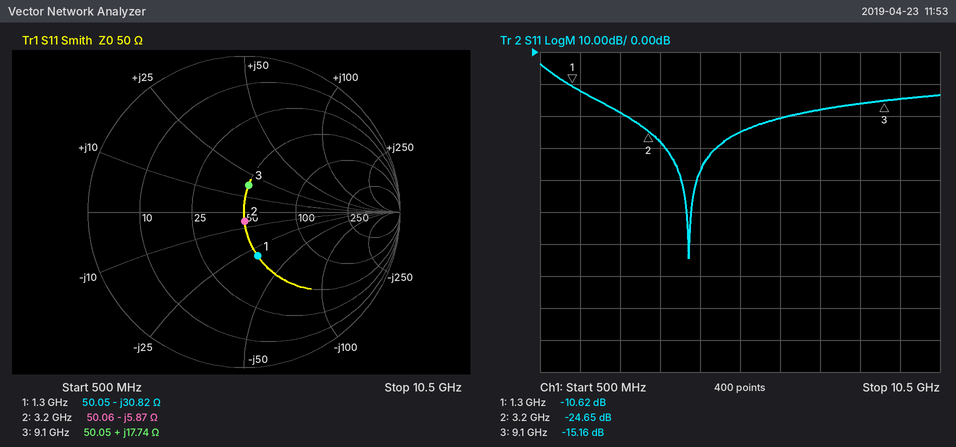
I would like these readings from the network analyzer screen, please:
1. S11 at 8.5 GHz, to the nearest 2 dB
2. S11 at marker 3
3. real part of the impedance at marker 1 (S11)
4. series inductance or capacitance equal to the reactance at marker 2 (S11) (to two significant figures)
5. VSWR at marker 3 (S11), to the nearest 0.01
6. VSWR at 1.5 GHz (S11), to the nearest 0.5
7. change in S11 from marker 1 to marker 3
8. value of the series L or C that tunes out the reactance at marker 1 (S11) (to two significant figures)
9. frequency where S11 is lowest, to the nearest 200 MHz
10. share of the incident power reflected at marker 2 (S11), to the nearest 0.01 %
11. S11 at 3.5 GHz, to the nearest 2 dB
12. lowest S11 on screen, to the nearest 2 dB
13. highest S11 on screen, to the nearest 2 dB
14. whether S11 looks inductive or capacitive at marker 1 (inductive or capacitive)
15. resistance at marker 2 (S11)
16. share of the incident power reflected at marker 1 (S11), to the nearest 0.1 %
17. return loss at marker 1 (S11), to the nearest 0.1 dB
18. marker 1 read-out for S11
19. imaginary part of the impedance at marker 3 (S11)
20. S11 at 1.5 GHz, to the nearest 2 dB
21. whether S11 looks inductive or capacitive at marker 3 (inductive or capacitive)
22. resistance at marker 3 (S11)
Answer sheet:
-16 dB
-15.16 dB
50.05 Ω
8.5 pF
1.42
1.5
-4.54 dB
3.8 nH
4.2 GHz
0.34 %
-28 dB
-64 dB
-4 dB
capacitive
50.06 Ω
8.7 %
10.6 dB
-10.62 dB
+17.74 Ω
-12 dB
inductive
50.05 Ω
